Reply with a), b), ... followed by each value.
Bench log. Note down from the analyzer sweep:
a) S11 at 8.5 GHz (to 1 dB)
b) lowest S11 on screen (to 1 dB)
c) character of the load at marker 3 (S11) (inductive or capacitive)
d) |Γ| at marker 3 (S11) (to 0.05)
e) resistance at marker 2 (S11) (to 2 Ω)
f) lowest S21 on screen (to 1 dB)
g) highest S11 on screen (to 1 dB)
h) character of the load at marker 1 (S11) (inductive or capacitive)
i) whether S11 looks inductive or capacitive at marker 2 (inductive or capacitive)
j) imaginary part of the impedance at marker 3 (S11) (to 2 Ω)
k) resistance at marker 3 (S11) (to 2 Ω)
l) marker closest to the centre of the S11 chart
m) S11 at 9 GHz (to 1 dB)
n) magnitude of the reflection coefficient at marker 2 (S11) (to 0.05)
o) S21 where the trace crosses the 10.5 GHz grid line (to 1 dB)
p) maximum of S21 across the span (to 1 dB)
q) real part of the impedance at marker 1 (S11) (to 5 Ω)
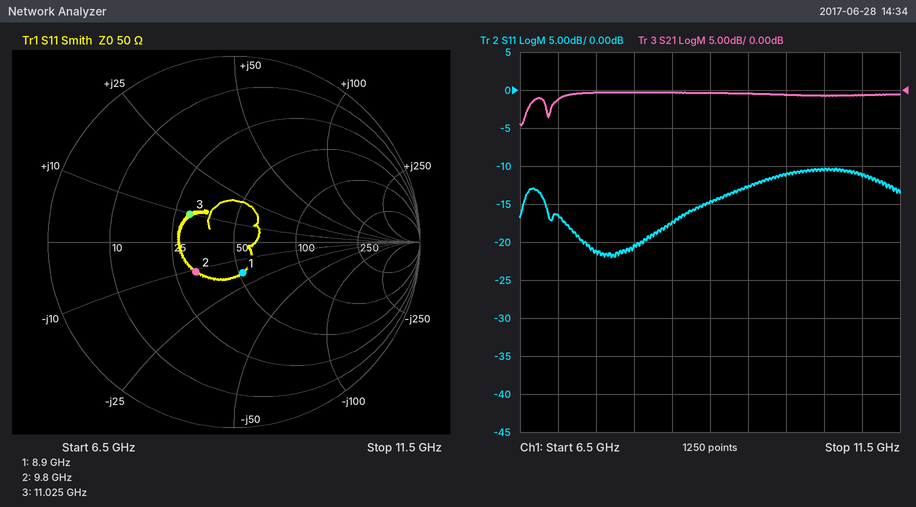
a) -17 dB
b) -22 dB
c) inductive
d) 0.30
e) 32 Ω
f) -5 dB
g) -10 dB
h) capacitive
i) capacitive
j) +10 Ω
k) 30 Ω
l) marker 1
m) -15 dB
n) 0.25
o) -1 dB
p) 0 dB
q) 50 Ω
